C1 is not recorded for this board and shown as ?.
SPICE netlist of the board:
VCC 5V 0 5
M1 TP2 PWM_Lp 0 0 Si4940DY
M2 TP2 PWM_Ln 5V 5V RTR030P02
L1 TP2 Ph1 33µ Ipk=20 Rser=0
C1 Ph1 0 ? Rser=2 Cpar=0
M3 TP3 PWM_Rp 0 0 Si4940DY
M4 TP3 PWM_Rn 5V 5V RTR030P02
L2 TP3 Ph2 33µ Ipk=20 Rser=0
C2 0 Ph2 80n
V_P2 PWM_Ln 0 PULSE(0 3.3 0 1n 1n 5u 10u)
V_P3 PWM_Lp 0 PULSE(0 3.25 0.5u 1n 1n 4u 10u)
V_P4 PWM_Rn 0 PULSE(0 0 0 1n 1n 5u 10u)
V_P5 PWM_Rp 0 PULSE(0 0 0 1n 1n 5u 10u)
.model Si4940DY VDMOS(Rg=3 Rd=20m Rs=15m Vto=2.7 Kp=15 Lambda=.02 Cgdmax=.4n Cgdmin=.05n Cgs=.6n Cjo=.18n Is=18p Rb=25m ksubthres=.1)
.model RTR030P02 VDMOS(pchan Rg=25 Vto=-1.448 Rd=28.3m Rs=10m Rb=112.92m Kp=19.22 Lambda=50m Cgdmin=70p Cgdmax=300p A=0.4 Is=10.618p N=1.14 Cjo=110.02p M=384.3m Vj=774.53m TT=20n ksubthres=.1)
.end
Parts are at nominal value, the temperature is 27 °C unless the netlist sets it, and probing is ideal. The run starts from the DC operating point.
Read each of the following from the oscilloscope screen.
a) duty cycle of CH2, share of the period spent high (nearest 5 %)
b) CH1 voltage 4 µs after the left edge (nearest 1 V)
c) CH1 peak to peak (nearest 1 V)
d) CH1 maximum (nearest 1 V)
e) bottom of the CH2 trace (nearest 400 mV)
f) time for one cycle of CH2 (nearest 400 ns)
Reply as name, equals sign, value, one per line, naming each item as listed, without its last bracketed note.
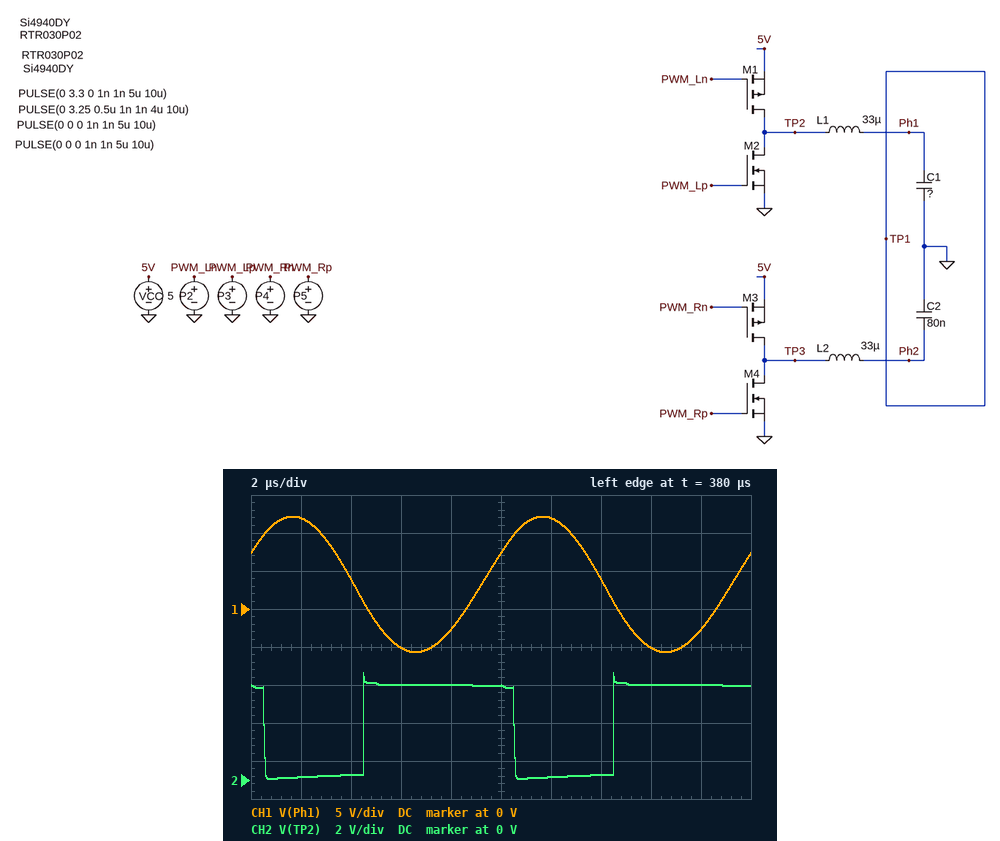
duty cycle of CH2, share of the period spent high = 60 %
CH1 voltage 4 µs after the left edge = 4 V
CH1 peak to peak = 18 V
CH1 maximum = 12 V
bottom of the CH2 trace = 0 V
time for one cycle of CH2 = 10.0 µs
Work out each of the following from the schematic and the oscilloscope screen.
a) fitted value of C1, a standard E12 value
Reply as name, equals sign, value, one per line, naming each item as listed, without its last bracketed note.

fitted value of C1, a standard E12 value = 100 nF
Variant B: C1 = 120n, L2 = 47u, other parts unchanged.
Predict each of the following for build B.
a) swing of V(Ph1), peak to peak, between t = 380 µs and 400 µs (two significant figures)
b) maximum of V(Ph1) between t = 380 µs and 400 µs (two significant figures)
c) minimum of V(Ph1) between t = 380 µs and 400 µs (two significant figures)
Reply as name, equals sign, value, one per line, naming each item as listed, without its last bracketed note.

swing of V(Ph1), peak to peak, between t = 380 µs and 400 µs = 10 V
maximum of V(Ph1) between t = 380 µs and 400 µs = 8.3 V
minimum of V(Ph1) between t = 380 µs and 400 µs = -1.8 V
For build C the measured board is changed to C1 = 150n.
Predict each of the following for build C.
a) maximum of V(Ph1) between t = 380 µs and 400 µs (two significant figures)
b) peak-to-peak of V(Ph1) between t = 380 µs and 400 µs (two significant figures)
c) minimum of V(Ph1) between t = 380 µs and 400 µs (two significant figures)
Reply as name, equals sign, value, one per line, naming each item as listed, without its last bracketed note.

maximum of V(Ph1) between t = 380 µs and 400 µs = 6.2 V
peak-to-peak of V(Ph1) between t = 380 µs and 400 µs = 6.1 V
minimum of V(Ph1) between t = 380 µs and 400 µs = 160 mV
